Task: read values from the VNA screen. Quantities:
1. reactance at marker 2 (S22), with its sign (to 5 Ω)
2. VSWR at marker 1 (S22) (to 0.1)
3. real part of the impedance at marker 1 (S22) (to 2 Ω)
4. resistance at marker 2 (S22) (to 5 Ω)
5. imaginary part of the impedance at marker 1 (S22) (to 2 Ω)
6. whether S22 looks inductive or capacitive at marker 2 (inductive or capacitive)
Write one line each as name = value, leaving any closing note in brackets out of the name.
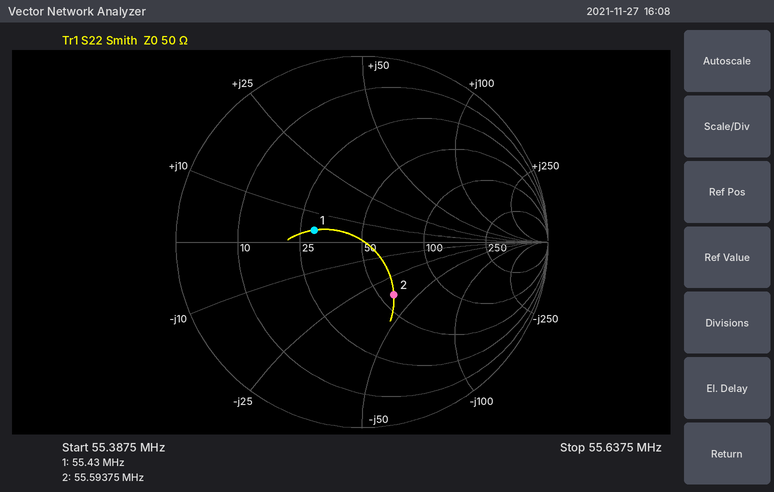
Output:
reactance at marker 2 (S22), with its sign = -35 Ω
VSWR at marker 1 (S22) = 1.7
real part of the impedance at marker 1 (S22) = 30 Ω
resistance at marker 2 (S22) = 60 Ω
imaginary part of the impedance at marker 1 (S22) = +4 Ω
whether S22 looks inductive or capacitive at marker 2 = capacitive
